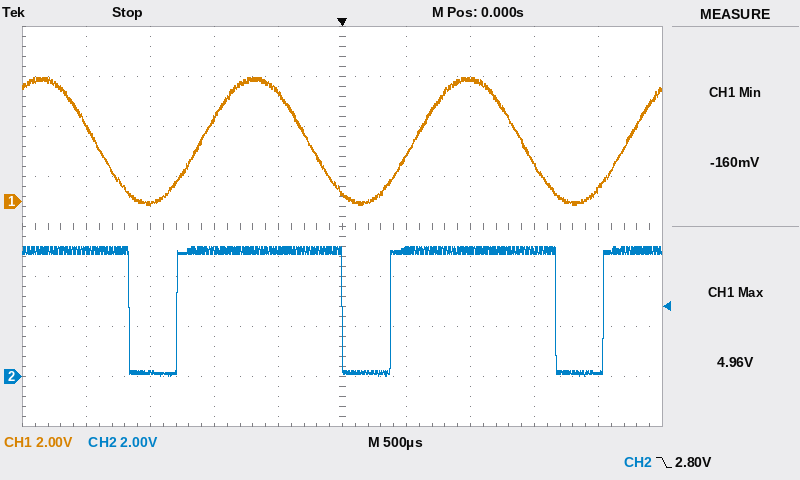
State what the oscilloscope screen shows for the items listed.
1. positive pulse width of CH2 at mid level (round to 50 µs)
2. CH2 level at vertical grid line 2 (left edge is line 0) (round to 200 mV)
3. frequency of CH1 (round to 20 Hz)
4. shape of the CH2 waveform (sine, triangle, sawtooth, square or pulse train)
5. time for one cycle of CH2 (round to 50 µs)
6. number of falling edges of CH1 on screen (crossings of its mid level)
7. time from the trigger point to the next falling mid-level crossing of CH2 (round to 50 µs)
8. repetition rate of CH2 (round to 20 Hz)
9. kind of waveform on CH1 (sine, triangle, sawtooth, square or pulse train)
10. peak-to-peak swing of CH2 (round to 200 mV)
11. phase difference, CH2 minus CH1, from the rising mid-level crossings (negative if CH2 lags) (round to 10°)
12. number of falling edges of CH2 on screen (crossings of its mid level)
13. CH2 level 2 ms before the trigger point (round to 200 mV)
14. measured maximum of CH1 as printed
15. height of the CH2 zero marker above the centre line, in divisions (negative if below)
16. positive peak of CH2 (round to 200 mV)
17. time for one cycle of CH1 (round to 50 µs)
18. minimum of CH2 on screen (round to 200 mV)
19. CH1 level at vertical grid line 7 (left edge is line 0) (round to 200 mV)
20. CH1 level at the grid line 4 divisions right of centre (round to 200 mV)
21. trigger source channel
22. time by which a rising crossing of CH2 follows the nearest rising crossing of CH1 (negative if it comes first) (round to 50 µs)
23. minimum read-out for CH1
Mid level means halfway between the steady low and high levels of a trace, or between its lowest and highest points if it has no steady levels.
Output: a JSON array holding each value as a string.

["1.30 ms", "200 mV", "600 Hz", "pulse train", "1.65 ms", "3", "1.65 ms", "600 Hz", "sine", "5.2 V", "+40°", "3", "5.0 V", "4.96 V", "-3.0 div", "5.2 V", "1.65 ms", "0.0 V", "4.8 V", "600 mV", "CH2", "-200 µs", "-160 mV"]
